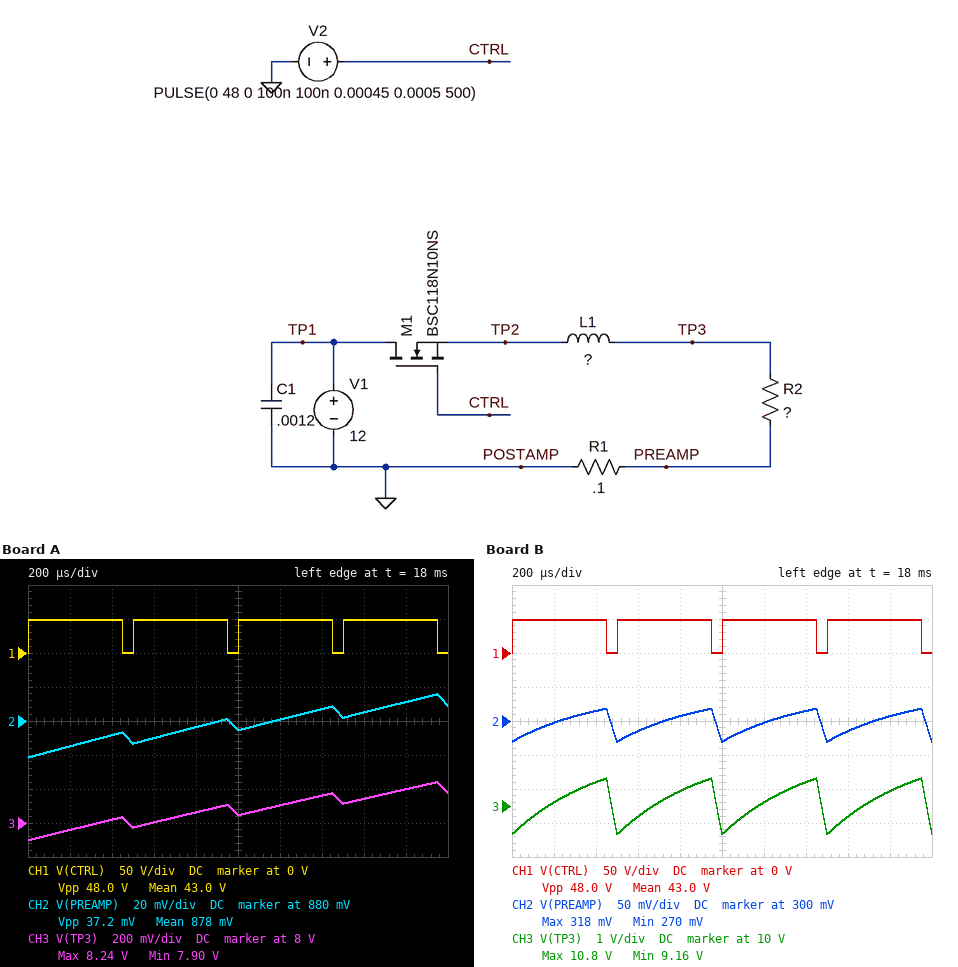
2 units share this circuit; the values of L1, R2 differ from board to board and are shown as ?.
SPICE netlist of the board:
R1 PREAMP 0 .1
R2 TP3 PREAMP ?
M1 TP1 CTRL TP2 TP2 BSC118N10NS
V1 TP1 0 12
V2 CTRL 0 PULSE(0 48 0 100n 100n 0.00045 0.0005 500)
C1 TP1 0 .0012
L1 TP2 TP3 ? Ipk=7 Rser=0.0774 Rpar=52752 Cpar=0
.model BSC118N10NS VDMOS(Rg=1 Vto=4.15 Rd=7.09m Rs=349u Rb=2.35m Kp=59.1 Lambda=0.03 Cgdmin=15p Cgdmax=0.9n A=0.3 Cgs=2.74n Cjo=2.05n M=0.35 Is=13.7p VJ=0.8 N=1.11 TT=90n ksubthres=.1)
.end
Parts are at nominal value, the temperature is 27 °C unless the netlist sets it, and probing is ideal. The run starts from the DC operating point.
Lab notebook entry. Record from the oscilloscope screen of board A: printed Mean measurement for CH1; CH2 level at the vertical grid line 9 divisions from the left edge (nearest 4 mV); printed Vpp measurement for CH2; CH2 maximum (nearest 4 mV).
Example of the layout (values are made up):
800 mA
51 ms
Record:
43.0 V
892 mV
37.2 mV
896 mV
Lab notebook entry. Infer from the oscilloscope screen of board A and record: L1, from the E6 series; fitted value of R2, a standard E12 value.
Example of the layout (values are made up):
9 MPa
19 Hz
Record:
10 mH
0.82 Ω
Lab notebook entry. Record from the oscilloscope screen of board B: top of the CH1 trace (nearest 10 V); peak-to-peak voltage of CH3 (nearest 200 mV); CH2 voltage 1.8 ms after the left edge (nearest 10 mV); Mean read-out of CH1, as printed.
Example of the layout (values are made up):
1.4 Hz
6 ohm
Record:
50 V
1.6 V
310 mV
43.0 V
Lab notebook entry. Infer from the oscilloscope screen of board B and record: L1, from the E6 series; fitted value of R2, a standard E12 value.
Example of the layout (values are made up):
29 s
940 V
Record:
1.5 mH
3.3 Ω
